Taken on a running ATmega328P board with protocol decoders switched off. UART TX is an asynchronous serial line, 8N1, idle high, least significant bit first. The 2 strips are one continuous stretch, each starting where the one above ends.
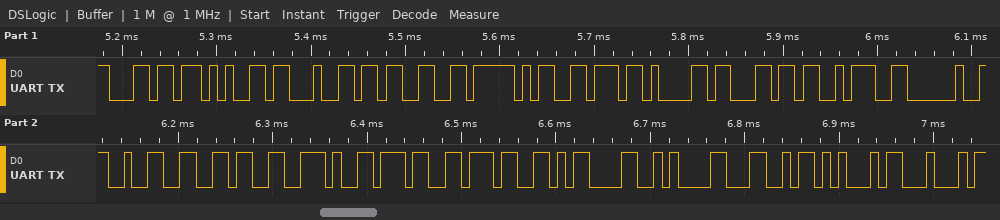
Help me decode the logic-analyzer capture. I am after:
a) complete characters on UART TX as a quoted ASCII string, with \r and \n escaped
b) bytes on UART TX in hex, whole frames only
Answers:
"led3_val: 26.77\r\nLED"
0x6C 0x65 0x64 0x33 0x5F 0x76 0x61 0x6C 0x3A 0x20 0x32 0x36 0x2E 0x37 0x37 0x0D 0x0A 0x4C 0x45 0x44
